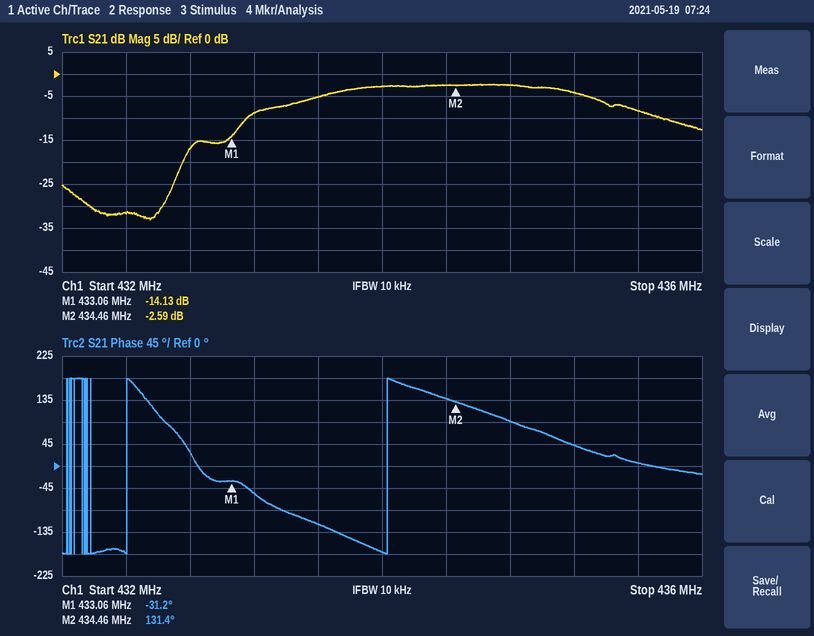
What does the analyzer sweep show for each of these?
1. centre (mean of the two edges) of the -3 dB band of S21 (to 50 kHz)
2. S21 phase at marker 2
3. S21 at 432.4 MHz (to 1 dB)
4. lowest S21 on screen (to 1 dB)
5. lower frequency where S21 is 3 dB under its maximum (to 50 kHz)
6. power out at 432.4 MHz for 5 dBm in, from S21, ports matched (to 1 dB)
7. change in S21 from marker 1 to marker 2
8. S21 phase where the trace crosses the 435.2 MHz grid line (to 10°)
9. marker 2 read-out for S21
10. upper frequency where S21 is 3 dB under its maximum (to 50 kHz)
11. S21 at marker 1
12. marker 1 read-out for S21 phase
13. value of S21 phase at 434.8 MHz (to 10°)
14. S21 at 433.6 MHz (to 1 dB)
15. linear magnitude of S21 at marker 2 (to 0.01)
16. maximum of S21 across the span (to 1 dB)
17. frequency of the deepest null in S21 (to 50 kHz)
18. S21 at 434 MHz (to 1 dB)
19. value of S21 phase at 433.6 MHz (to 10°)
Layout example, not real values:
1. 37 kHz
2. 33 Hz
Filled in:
1. 434.45 MHz
2. 131.4°
3. -32 dB
4. -33 dB
5. 433.60 MHz
6. -27 dBm
7. 11.54 dB
8. 40°
9. -2.59 dB
10. 435.30 MHz
11. -14.13 dB
12. -31.2°
13. 90°
14. -5 dB
15. 0.74
16. -2 dB
17. 432.55 MHz
18. -3 dB
19. -120°
